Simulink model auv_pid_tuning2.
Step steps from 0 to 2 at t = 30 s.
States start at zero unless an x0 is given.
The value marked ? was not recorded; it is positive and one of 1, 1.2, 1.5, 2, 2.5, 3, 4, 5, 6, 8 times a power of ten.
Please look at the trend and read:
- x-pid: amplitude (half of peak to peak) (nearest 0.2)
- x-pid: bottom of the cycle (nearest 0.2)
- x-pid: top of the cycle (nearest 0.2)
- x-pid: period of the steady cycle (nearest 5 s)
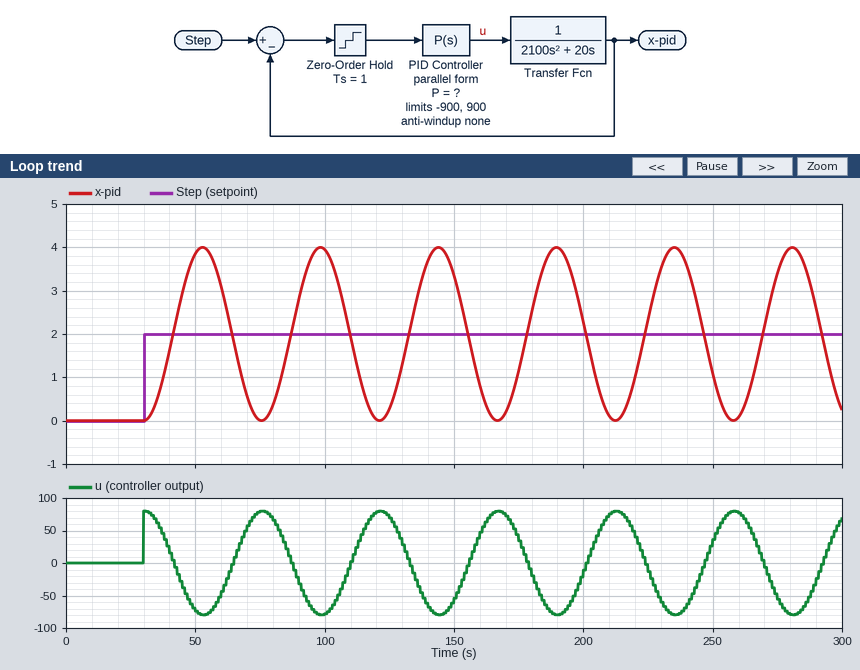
2.0
0.0
4.0
45 s
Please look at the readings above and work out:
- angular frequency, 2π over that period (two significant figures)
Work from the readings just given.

0.14 rad/s
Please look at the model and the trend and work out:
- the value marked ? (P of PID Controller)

40
